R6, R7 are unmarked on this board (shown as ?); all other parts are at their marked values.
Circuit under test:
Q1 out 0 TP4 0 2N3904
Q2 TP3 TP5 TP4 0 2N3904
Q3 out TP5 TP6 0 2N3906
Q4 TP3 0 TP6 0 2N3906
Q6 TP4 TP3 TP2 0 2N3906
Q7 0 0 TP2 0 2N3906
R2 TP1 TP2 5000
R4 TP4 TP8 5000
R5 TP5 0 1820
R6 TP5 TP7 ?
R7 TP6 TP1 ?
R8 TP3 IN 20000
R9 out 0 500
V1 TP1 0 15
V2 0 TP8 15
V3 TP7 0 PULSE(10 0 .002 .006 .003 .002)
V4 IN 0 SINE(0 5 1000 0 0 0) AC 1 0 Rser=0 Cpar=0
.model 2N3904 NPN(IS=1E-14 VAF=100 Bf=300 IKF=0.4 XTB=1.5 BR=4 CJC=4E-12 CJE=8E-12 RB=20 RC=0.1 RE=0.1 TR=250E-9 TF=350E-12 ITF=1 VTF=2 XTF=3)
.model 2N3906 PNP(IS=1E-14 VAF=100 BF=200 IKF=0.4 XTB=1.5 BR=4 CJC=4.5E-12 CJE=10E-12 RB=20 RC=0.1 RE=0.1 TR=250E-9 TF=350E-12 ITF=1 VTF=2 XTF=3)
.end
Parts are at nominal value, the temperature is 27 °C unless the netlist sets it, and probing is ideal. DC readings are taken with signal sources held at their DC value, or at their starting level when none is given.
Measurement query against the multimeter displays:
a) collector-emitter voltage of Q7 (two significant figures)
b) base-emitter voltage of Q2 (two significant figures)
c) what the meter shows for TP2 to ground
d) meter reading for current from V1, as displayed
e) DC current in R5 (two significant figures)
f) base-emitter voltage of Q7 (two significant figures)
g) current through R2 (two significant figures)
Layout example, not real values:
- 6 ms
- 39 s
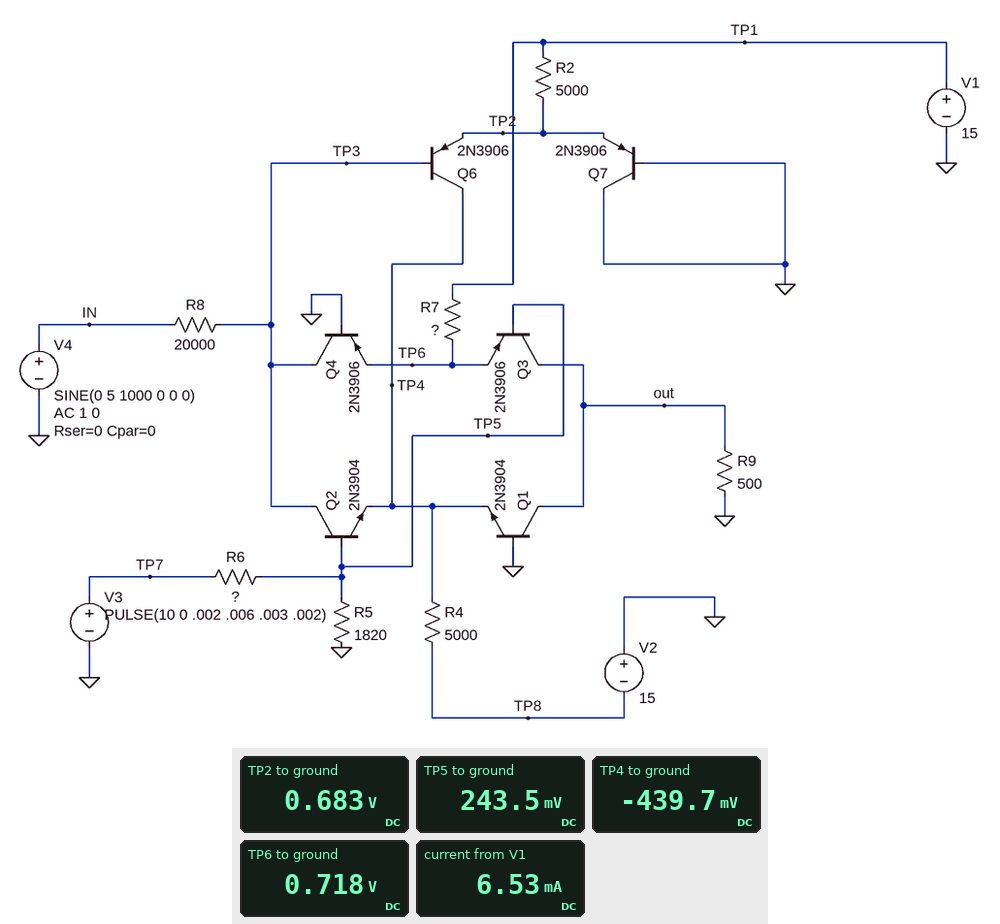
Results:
- -680 mV
- 680 mV
- 0.683 V
- 6.53 mA
- 130 µA
- -680 mV
- 2.9 mA
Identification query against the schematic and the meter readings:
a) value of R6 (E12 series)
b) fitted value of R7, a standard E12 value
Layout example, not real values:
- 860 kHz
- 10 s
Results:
- 68 kΩ
- 3.9 kΩ
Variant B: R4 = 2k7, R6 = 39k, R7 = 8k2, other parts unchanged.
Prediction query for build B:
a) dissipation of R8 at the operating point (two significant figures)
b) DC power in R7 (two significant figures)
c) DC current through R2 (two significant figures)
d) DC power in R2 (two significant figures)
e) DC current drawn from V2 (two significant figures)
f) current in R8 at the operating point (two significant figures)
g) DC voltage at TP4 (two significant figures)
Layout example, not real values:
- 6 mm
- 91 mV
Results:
- 19 µW
- 25 mW
- 3.0 mA
- 45 mW
- 5.3 mA
- 31 µA
- -640 mV
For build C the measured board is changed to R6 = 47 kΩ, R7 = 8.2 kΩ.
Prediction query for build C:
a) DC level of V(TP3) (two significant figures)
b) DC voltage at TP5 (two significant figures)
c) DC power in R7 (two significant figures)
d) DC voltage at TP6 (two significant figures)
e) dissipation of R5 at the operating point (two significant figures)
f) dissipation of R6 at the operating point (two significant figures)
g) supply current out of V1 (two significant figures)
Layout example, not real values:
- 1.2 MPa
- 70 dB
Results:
- 8.9 mV
- 360 mV
- 25 mW
- 670 mV
- 72 µW
- 2.0 mW
- 4.6 mA
